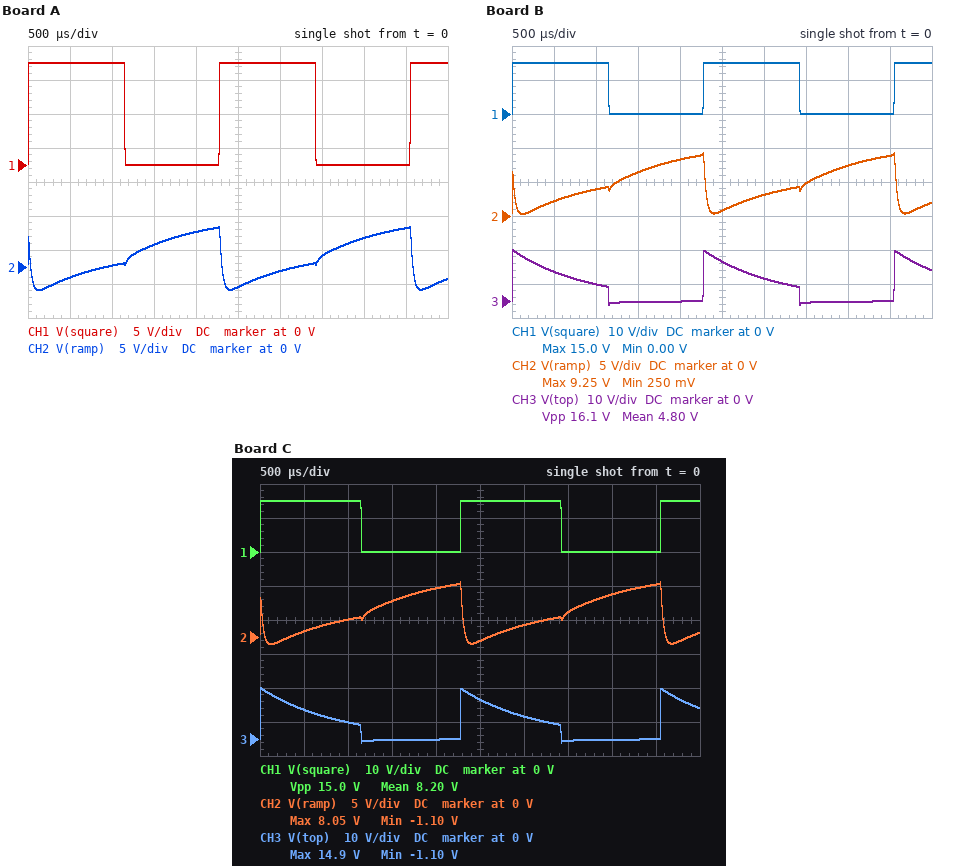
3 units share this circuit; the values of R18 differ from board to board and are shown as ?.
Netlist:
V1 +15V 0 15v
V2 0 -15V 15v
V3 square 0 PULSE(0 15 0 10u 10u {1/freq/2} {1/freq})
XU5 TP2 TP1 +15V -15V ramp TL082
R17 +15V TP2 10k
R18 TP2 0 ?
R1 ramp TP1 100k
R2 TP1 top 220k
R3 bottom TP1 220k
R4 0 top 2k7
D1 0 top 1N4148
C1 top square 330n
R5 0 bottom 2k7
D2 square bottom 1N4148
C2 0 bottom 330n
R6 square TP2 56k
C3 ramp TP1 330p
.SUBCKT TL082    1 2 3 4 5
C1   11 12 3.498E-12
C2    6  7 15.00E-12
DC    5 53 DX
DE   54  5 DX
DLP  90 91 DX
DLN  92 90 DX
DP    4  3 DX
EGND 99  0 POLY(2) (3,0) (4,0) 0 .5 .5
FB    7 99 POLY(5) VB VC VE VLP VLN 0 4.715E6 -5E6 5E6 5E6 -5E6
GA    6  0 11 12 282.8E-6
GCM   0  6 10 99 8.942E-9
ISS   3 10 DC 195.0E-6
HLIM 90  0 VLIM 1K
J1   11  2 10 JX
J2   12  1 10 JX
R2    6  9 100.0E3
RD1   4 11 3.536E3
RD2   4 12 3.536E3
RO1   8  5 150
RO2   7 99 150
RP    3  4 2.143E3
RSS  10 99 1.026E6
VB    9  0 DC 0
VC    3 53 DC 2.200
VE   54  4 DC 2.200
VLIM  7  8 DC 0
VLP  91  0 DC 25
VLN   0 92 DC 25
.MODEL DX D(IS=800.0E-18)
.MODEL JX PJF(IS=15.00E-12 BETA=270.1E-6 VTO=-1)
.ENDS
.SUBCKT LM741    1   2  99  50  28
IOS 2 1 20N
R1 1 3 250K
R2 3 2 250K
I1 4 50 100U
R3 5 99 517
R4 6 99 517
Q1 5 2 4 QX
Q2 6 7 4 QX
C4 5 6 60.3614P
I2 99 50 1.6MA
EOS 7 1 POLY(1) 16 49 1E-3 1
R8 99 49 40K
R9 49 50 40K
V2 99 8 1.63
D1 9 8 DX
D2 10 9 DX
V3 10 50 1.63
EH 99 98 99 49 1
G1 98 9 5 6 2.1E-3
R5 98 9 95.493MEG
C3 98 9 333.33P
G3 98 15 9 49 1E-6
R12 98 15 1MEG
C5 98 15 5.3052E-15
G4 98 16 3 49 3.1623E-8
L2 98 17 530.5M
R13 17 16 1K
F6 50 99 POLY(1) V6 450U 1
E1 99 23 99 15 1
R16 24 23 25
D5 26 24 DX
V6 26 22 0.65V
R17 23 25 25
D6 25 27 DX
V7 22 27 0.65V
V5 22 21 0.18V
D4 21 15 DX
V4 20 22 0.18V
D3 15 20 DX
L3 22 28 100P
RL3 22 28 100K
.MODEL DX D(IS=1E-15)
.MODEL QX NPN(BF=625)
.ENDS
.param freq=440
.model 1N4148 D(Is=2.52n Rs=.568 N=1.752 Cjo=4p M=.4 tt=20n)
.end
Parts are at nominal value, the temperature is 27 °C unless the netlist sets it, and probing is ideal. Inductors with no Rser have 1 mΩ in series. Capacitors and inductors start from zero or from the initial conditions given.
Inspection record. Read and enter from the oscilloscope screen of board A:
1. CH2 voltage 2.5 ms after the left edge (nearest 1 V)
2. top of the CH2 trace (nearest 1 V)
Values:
-3 V
6 V
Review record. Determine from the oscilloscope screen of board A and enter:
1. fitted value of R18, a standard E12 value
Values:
3.9 kΩ
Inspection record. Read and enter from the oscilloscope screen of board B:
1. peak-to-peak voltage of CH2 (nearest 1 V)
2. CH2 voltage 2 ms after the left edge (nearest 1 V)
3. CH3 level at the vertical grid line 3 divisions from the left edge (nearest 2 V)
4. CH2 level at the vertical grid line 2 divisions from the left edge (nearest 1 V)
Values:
9 V
8 V
0 V
4 V
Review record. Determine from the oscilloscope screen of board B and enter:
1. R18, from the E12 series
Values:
6.8 kΩ
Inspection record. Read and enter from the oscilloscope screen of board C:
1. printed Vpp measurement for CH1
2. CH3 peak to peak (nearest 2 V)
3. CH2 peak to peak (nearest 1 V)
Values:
15.0 V
16 V
9 V
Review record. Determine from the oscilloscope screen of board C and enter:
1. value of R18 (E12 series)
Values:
5.6 kΩ
